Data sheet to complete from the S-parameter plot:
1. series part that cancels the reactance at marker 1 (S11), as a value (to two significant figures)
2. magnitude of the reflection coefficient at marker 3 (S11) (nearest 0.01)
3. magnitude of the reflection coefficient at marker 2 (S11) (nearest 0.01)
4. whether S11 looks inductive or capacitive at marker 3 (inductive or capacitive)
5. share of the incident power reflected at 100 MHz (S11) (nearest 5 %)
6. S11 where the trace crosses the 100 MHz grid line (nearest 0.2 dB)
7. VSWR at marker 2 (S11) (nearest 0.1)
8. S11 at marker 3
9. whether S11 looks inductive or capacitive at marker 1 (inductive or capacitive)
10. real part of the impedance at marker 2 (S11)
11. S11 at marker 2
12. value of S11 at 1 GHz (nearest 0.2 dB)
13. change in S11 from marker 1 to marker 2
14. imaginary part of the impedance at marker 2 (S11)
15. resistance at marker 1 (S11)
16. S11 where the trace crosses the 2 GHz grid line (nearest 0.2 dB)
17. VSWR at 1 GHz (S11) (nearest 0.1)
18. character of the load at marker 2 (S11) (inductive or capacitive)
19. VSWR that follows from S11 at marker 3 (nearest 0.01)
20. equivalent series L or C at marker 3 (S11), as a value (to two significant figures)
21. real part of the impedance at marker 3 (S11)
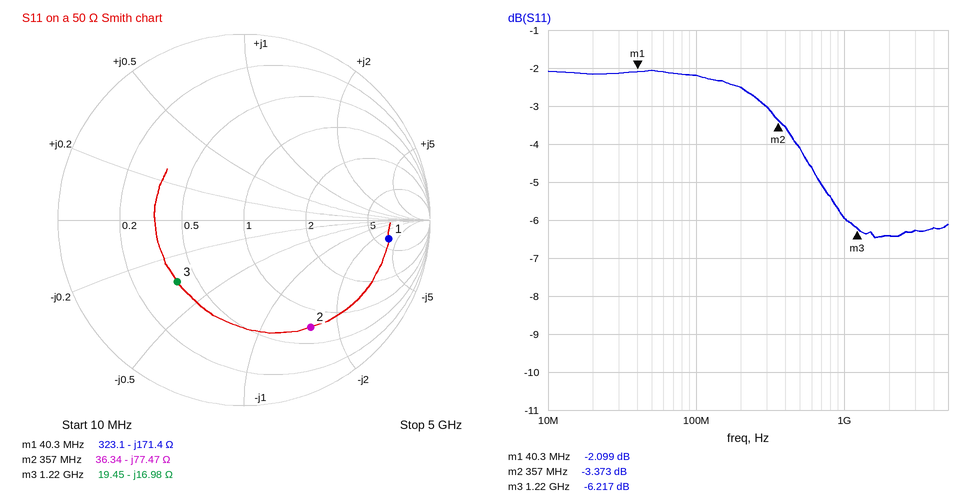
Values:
680 nH
0.49
0.68
capacitive
60 %
-2.2 dB
5.2
-6.217 dB
capacitive
36.34 Ω
-3.373 dB
-6.0 dB
-1.274 dB
-77.47 Ω
323.1 Ω
-6.4 dB
3.0
capacitive
2.91
7.7 pF
19.45 Ω
